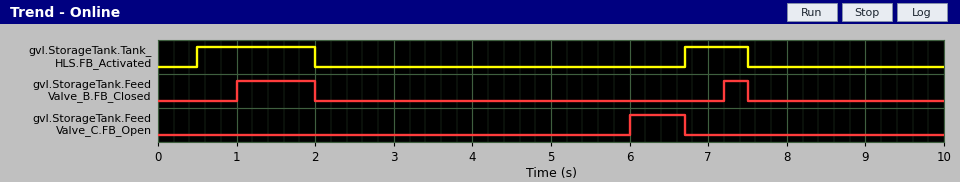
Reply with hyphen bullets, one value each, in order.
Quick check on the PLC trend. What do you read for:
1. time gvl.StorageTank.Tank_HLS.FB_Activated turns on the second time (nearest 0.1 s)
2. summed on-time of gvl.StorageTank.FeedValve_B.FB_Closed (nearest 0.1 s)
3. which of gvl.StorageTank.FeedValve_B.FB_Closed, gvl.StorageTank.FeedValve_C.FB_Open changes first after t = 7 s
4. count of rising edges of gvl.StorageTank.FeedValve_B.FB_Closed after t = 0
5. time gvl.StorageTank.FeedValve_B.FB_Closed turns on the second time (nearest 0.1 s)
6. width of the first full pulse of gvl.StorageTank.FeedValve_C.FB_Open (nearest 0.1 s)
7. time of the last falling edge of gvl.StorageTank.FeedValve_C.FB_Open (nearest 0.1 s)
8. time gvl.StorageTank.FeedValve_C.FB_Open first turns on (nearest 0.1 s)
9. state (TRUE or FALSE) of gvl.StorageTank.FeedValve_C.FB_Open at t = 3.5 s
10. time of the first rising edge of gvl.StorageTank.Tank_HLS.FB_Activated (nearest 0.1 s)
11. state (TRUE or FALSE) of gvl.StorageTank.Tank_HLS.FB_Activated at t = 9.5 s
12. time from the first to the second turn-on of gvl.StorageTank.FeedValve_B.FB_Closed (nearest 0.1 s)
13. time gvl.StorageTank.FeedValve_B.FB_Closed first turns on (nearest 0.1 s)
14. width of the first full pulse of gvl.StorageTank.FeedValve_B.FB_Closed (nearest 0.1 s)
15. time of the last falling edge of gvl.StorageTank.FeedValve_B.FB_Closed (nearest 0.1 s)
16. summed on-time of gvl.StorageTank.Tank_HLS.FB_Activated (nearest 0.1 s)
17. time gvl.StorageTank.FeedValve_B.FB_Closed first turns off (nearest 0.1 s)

- 6.7 s
- 1.3 s
- gvl.StorageTank.FeedValve_B.FB_Closed
- 2
- 7.2 s
- 0.7 s
- 6.7 s
- 6.0 s
- FALSE
- 0.5 s
- FALSE
- 6.2 s
- 1.0 s
- 1.0 s
- 7.5 s
- 2.3 s
- 2.0 s
